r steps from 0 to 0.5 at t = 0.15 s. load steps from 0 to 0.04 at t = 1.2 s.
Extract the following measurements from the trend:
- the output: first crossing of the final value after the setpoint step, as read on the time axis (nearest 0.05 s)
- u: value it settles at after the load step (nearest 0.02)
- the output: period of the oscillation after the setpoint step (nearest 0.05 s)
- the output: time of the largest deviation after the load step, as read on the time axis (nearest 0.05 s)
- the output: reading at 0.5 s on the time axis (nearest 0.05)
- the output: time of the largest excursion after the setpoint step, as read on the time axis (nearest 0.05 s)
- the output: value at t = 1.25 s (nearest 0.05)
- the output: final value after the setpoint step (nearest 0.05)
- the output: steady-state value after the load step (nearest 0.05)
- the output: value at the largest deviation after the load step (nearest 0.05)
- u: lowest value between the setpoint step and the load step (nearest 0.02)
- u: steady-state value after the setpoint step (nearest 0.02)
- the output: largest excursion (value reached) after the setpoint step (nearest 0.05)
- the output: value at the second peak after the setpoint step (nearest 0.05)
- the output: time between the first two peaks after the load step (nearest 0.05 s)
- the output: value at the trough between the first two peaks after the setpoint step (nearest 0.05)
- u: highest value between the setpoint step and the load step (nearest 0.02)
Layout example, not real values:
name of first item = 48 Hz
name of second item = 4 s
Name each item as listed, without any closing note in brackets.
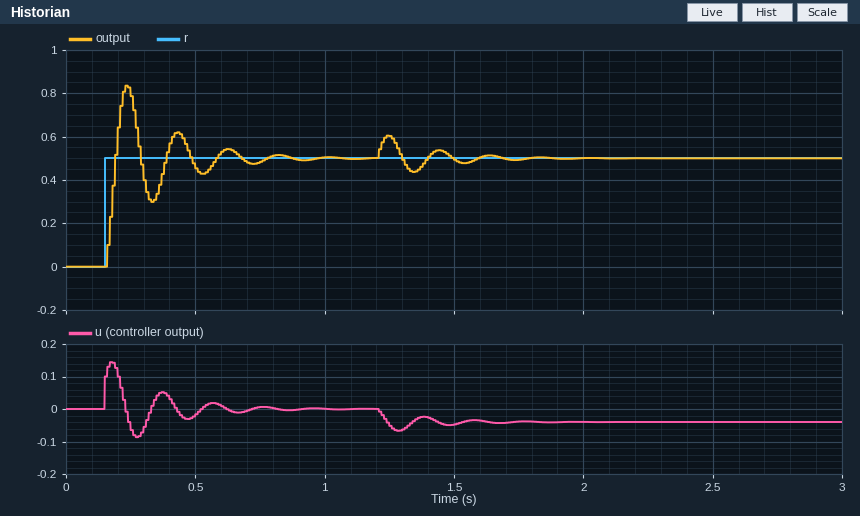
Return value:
the output: first crossing of the final value after the setpoint step, as read on the time axis = 0.20 s
u: value it settles at after the load step = -0.04
the output: period of the oscillation after the setpoint step = 0.20 s
the output: time of the largest deviation after the load step, as read on the time axis = 1.25 s
the output: reading at 0.5 s on the time axis = 0.45
the output: time of the largest excursion after the setpoint step, as read on the time axis = 0.25 s
the output: value at t = 1.25 s = 0.60
the output: final value after the setpoint step = 0.50
the output: steady-state value after the load step = 0.50
the output: value at the largest deviation after the load step = 0.60
u: lowest value between the setpoint step and the load step = -0.08
u: steady-state value after the setpoint step = 0.00
the output: largest excursion (value reached) after the setpoint step = 0.85
the output: value at the second peak after the setpoint step = 0.60
the output: time between the first two peaks after the load step = 0.20 s
the output: value at the trough between the first two peaks after the setpoint step = 0.30
u: highest value between the setpoint step and the load step = 0.14
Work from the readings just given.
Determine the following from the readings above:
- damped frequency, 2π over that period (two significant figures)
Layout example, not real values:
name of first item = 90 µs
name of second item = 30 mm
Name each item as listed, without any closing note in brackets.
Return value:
damped frequency, 2π over that period = 31 rad/s
